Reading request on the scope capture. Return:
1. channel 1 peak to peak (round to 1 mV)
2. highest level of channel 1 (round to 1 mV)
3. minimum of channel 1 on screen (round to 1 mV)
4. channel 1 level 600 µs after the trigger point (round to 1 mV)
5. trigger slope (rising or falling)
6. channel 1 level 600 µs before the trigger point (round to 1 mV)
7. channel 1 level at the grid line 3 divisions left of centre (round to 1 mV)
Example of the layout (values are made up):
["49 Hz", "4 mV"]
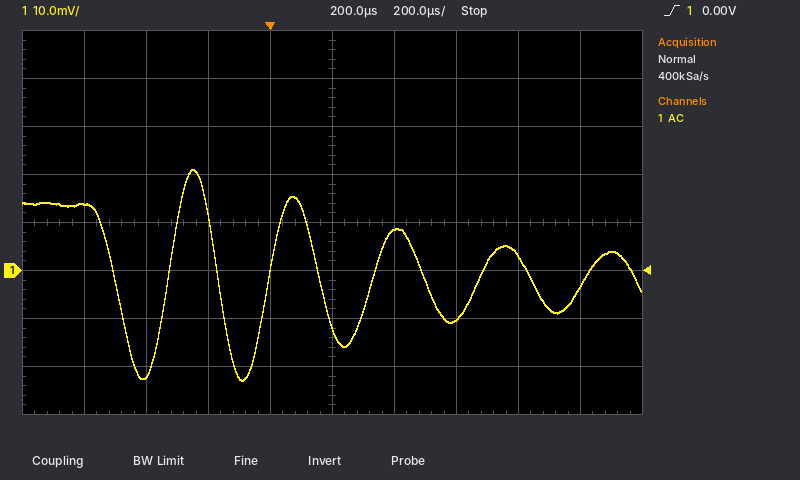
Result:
["44 mV", "21 mV", "-23 mV", "-10 mV", "rising", "14 mV", "-22 mV"]
